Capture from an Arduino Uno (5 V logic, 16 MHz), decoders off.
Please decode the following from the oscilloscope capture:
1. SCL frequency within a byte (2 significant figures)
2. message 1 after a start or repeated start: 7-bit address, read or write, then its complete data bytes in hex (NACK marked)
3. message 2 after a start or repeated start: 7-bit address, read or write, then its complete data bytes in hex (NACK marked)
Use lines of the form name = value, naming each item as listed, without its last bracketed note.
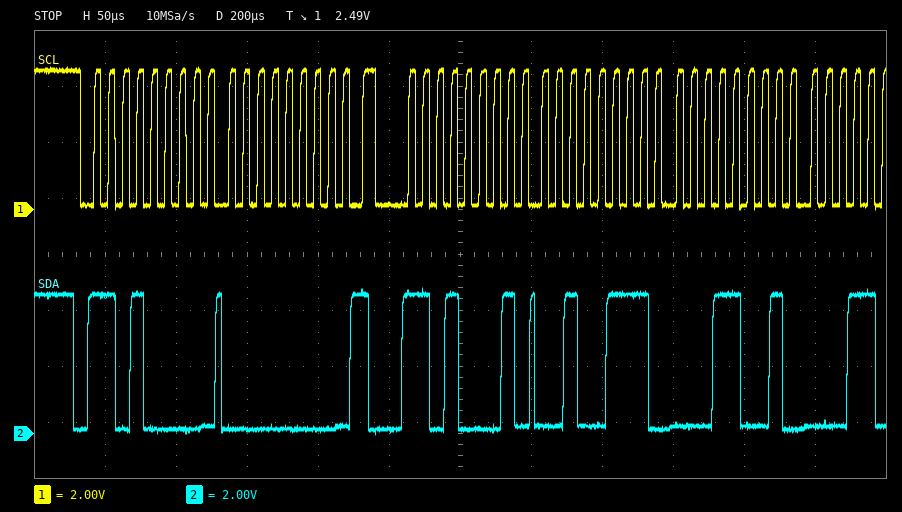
SCL frequency within a byte = 100 kHz
message 1 after a start or repeated start: 7-bit address, read or write, then its complete data bytes in hex = 0x68 write: 00
message 2 after a start or repeated start: 7-bit address, read or write, then its complete data bytes in hex = 0x68 read: 27 19
